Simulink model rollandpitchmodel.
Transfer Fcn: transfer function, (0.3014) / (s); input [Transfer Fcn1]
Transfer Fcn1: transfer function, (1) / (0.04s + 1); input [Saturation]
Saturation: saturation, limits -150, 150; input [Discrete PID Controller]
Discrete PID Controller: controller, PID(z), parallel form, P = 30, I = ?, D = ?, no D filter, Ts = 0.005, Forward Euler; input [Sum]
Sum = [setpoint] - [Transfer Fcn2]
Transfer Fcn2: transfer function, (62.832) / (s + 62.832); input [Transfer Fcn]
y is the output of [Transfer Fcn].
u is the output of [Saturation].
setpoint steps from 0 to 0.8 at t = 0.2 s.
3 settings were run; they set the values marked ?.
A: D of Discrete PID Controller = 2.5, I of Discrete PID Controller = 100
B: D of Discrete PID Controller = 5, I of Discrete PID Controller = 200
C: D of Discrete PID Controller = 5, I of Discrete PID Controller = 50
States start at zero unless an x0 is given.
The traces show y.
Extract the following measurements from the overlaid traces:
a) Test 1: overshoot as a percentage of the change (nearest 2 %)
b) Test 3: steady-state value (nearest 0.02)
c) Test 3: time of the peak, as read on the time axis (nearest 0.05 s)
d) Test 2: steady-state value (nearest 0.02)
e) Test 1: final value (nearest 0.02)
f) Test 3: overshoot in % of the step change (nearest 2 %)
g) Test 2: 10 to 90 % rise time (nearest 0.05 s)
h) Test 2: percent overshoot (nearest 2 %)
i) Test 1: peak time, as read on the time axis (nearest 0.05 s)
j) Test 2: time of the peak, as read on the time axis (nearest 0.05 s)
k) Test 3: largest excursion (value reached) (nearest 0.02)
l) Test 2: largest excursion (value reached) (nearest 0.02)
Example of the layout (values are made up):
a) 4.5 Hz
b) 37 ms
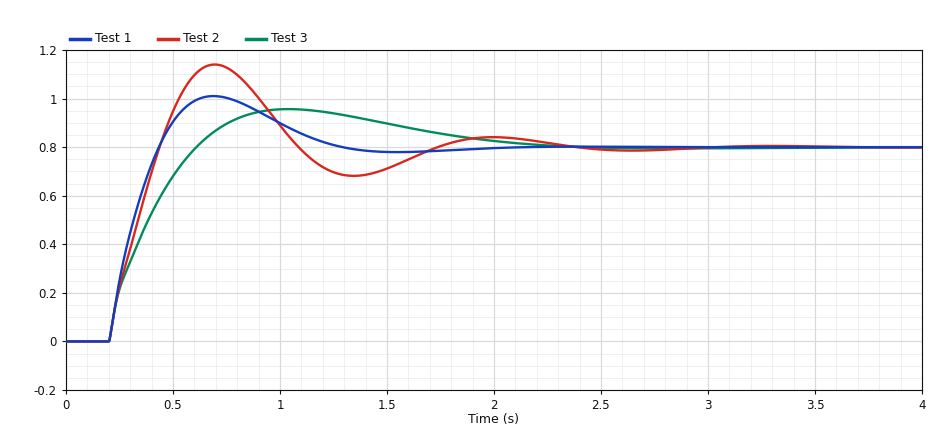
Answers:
a) 26 %
b) 0.80
c) 1.05 s
d) 0.80
e) 0.80
f) 20 %
g) 0.20 s
h) 42 %
i) 0.70 s
j) 0.70 s
k) 0.96
l) 1.14
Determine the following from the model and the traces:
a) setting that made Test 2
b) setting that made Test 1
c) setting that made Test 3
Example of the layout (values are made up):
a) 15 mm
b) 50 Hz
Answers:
a) B
b) A
c) C
